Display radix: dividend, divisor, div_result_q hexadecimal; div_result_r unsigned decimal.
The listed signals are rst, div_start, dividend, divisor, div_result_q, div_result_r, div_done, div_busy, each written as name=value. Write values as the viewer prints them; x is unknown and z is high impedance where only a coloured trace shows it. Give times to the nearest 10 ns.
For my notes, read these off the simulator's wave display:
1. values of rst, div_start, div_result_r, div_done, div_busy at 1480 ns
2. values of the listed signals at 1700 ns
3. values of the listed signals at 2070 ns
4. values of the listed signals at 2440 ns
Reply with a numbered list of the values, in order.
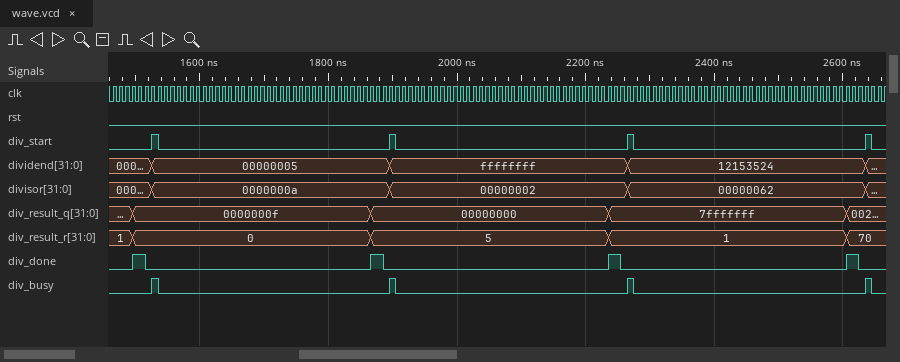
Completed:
1. rst=0, div_start=0, div_result_r=1, div_done=0, div_busy=0
2. rst=0, div_start=0, dividend=00000005, divisor=0000000a, div_result_q=0000000f, div_result_r=0, div_done=0, div_busy=0
3. rst=0, div_start=0, dividend=ffffffff, divisor=00000002, div_result_q=00000000, div_result_r=5, div_done=0, div_busy=0
4. rst=0, div_start=0, dividend=12153524, divisor=00000062, div_result_q=7fffffff, div_result_r=1, div_done=0, div_busy=0
